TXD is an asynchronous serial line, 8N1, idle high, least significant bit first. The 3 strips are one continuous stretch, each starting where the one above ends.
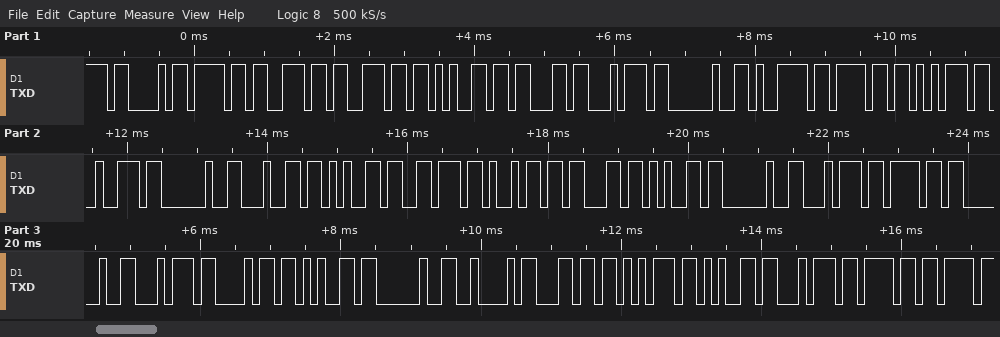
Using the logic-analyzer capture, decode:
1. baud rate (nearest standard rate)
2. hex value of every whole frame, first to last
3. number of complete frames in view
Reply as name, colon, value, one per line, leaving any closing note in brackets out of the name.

baud rate: 9600 baud
hex value of every whole frame, first to last: 43 6F 6E 6E 65 63 74 20 79 6F 75 72 20 64 65 76 69 63 65 20 74 6F 20 74 68 65 20 42 6C 75 65 74 6F
number of complete frames in view: 33
